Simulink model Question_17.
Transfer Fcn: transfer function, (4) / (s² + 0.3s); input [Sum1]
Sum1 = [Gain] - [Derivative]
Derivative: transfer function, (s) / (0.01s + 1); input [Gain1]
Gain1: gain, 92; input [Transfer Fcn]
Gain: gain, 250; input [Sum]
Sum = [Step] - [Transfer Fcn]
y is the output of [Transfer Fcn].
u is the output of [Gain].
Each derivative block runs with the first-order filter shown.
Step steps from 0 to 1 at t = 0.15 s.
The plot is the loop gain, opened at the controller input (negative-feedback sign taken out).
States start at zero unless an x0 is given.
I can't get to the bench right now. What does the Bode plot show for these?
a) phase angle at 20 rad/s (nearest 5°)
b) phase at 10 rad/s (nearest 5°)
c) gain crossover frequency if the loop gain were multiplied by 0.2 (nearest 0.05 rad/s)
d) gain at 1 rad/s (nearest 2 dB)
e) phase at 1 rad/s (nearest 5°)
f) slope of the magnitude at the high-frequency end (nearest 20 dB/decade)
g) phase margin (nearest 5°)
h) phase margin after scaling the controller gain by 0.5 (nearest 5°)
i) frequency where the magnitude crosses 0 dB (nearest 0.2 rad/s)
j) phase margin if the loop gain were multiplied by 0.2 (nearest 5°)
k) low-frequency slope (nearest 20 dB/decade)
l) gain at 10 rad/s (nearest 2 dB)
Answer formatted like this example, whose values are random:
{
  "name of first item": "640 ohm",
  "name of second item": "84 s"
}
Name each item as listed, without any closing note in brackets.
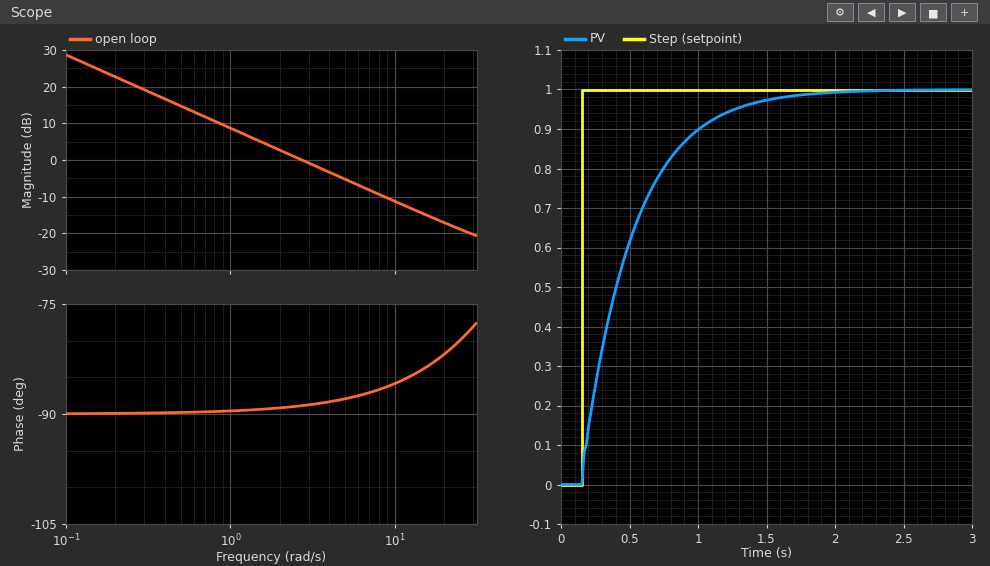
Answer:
{
  "phase angle at 20 rad/s": "-80°",
  "phase at 10 rad/s": "-85°",
  "gain crossover frequency if the loop gain were multiplied by 0.2": "0.55 rad/s",
  "gain at 1 rad/s": "8 dB",
  "phase at 1 rad/s": "-90°",
  "slope of the magnitude at the high-frequency end": "-20 dB/decade",
  "phase margin": "90°",
  "phase margin after scaling the controller gain by 0.5": "90°",
  "frequency where the magnitude crosses 0 dB": "2.8 rad/s",
  "phase margin if the loop gain were multiplied by 0.2": "90°",
  "low-frequency slope": "-20 dB/decade",
  "gain at 10 rad/s": "-12 dB"
}
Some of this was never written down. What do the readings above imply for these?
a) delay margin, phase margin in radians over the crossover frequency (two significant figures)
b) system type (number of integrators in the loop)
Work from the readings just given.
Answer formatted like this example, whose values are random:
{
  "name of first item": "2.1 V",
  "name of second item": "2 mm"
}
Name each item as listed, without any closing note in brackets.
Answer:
{
  "delay margin, phase margin in radians over the crossover frequency": "0.56 s",
  "system type": "1"
}
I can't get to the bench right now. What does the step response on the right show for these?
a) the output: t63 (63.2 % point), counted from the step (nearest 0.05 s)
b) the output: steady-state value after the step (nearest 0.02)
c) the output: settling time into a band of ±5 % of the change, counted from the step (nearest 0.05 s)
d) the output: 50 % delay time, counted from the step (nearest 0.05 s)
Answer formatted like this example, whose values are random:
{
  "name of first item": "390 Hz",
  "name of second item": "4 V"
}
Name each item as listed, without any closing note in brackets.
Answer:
{
  "the output: t63 (63.2 % point), counted from the step": "0.35 s",
  "the output: steady-state value after the step": "1.00",
  "the output: settling time into a band of ±5 % of the change, counted from the step": "1.10 s",
  "the output: 50 % delay time, counted from the step": "0.25 s"
}
